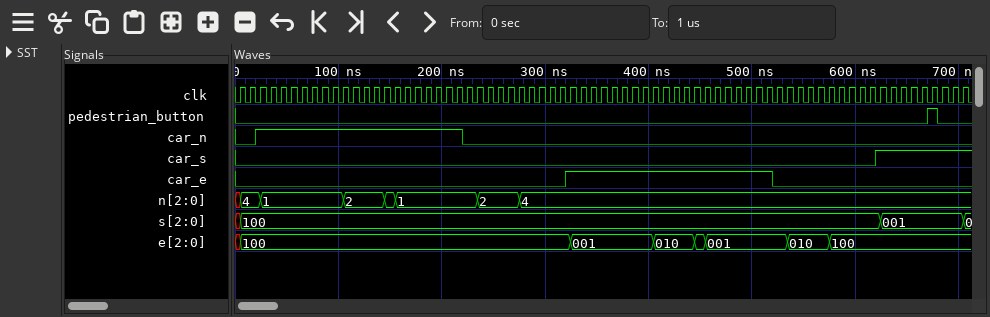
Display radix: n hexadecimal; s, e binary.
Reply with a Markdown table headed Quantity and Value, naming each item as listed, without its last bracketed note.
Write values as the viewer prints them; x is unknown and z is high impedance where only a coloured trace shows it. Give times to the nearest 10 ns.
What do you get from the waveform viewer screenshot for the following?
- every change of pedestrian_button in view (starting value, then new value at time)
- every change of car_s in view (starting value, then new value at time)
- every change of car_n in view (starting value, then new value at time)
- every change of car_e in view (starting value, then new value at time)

| Quantity | Value |
|---|---|
| every change of pedestrian_button in view | 0, 1 at 670 ns, 0 at 680 ns |
| every change of car_s in view | 0, 1 at 620 ns |
| every change of car_n in view | 0, 1 at 20 ns, 0 at 220 ns |
| every change of car_e in view | 0, 1 at 320 ns, 0 at 520 ns |
